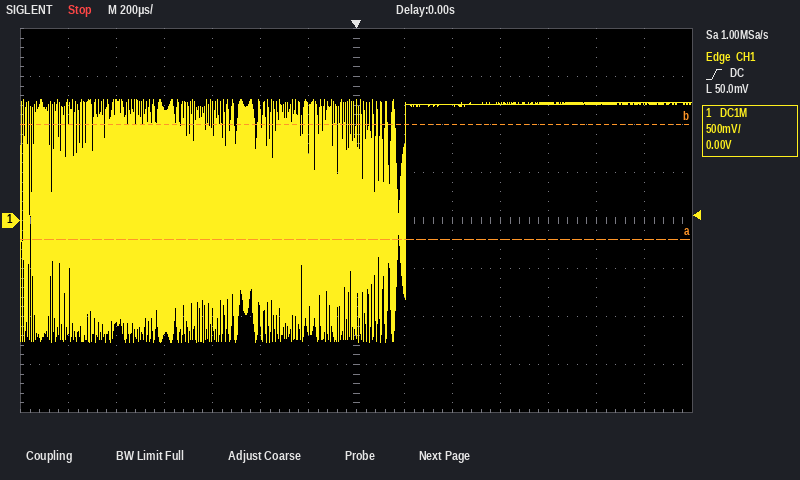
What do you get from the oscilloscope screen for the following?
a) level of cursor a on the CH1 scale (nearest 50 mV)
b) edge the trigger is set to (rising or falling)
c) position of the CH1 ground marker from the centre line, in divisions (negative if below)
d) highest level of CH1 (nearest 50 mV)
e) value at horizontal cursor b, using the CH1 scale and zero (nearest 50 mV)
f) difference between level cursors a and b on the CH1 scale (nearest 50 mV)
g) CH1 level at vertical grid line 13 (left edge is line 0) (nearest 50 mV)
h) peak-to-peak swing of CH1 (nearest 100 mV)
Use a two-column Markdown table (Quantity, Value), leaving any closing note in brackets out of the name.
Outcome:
| Quantity | Value |
|---|---|
| level of cursor a on the CH1 scale | -200 mV |
| edge the trigger is set to | rising |
| position of the CH1 ground marker from the centre line, in divisions | 0.0 div |
| highest level of CH1 | 1.25 V |
| value at horizontal cursor b, using the CH1 scale and zero | 1.00 V |
| difference between level cursors a and b on the CH1 scale | 1.20 V |
| CH1 level at vertical grid line 13 (left edge is line 0) | 1.20 V |
| peak-to-peak swing of CH1 | 2.50 V |
